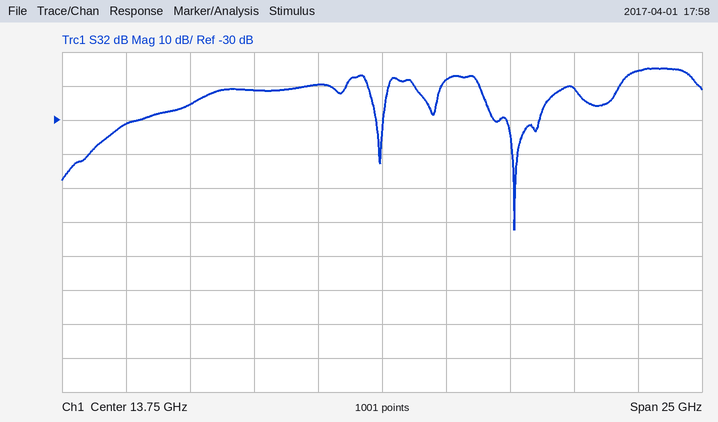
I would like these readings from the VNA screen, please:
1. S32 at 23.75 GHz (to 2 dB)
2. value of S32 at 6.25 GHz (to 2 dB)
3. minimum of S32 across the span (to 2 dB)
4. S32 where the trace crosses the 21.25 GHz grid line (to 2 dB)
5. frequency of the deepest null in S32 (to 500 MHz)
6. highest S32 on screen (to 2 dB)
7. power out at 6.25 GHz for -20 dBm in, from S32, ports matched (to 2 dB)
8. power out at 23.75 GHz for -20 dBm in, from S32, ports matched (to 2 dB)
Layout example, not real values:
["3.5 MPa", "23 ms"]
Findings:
["-16 dB", "-26 dB", "-62 dB", "-20 dB", "19.0 GHz", "-14 dB", "-46 dBm", "-36 dBm"]
